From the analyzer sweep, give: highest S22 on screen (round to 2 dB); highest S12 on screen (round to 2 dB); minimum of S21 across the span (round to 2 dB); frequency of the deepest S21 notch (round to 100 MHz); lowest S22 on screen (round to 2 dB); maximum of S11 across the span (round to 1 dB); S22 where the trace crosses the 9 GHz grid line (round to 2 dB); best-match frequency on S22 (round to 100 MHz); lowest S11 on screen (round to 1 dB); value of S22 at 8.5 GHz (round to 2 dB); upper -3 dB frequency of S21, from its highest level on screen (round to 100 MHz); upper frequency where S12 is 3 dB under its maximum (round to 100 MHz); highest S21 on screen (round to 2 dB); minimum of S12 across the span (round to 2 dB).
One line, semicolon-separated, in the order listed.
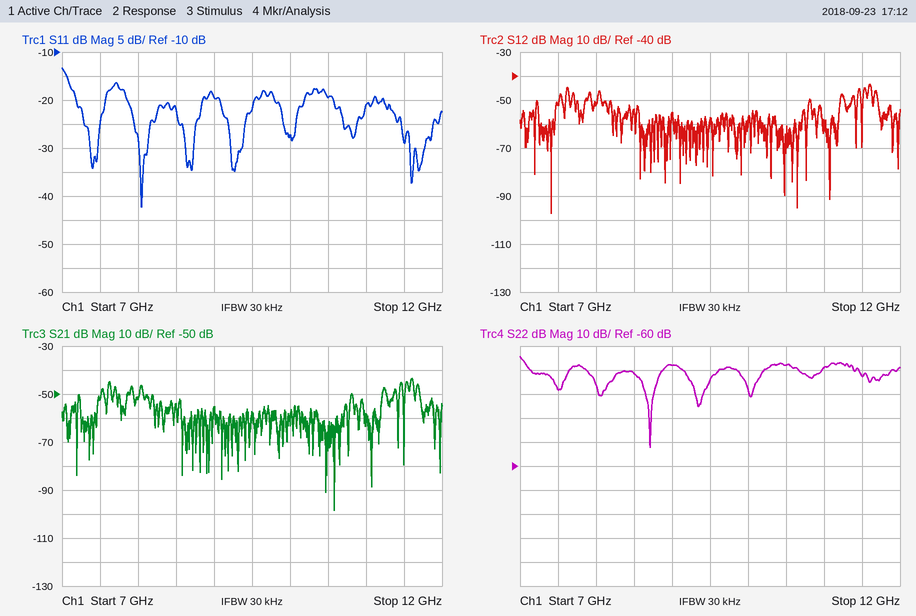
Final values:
-14 dB; -44 dB; -98 dB; 10.6 GHz; -52 dB; -13 dB; -18 dB; 8.7 GHz; -42 dB; -22 dB; 11.6 GHz; 11.6 GHz; -44 dB; -98 dB
